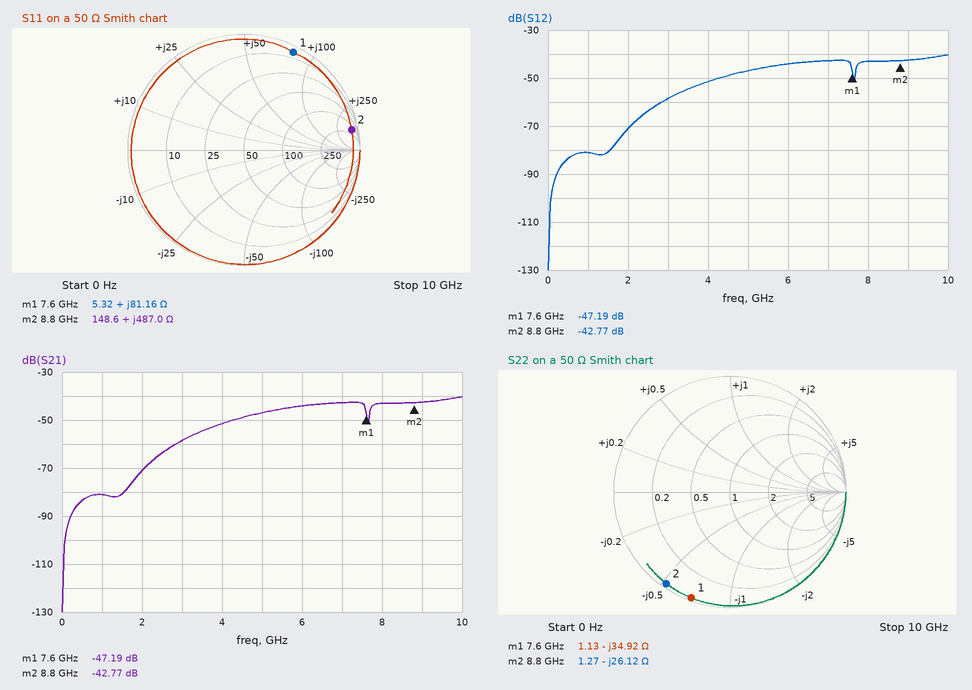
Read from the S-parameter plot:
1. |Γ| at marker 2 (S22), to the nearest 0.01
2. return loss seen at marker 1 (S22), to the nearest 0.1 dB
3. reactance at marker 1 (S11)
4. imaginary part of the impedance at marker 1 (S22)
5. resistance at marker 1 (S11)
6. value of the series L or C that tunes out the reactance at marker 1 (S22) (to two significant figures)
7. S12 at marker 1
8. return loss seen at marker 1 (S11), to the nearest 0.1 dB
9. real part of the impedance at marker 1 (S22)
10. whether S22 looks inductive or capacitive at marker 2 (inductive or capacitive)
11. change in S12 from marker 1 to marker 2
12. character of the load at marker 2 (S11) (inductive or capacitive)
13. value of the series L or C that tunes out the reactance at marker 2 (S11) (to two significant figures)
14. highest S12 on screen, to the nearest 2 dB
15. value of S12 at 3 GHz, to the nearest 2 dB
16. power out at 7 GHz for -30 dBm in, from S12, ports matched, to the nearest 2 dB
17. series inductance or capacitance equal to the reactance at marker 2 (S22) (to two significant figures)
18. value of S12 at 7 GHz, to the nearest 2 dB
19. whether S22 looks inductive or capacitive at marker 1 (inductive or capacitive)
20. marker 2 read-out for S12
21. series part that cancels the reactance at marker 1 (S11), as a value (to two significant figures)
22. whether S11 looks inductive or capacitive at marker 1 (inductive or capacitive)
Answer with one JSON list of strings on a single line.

["0.96", "0.3 dB", "+81.16 Ω", "-34.92 Ω", "5.32 Ω", "730 pH", "-47.19 dB", "0.5 dB", "1.13 Ω", "capacitive", "4.42 dB", "inductive", "37 fF", "-40 dB", "-58 dB", "-72 dBm", "690 fF", "-42 dB", "capacitive", "-42.77 dB", "260 fF", "inductive"]
